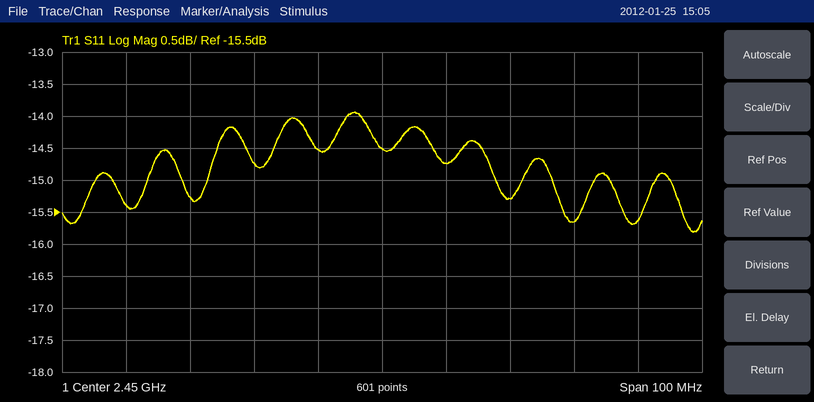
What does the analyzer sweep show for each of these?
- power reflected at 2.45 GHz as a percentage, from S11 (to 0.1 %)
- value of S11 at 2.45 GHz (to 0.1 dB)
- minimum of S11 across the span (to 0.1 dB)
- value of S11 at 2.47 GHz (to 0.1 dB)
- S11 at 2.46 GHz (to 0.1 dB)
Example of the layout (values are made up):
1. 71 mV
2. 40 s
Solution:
1. 3.5 %
2. -14.5 dB
3. -15.8 dB
4. -15.3 dB
5. -14.7 dB
